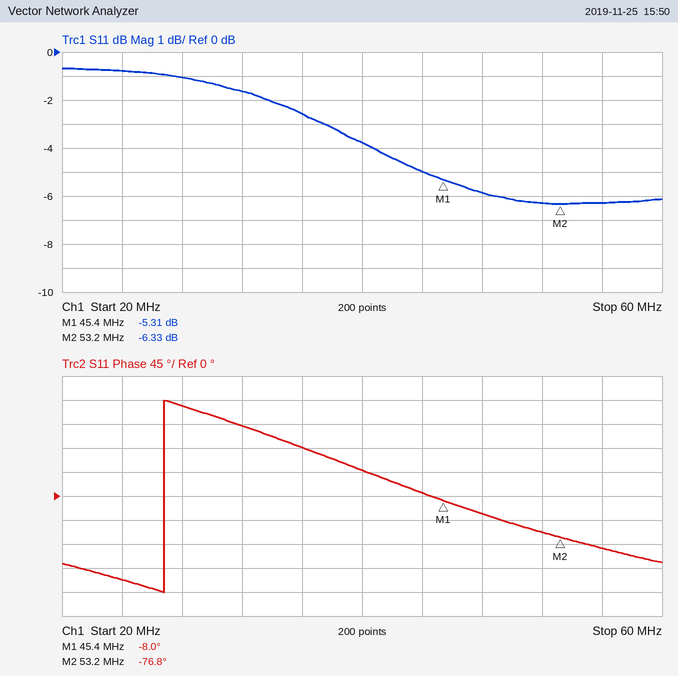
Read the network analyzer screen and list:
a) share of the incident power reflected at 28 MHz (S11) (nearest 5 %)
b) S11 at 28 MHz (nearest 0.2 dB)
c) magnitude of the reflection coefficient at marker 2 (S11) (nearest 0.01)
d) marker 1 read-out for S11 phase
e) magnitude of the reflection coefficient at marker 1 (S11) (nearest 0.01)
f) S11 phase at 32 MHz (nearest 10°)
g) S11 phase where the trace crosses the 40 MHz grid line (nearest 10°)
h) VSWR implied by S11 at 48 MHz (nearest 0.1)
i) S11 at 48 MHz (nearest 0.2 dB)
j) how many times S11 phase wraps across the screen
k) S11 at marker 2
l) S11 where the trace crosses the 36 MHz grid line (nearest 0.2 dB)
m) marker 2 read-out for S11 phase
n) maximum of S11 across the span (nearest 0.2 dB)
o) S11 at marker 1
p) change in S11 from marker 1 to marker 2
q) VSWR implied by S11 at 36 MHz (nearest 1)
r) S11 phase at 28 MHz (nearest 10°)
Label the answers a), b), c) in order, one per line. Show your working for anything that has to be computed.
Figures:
a) 10^(-1/10) ≈ 79.4 %, so 80 % to the nearest 5 %
b) -1.0 dB
c) 10^(-6.33/20) ≈ 0.48
d) -8.0°
e) 10^(-5.31/20) ≈ 0.54
f) 130°
g) 50°
h) |Γ| = 10^(-5.8/20) = 0.5129; VSWR = (1 + 0.5129)/(1 − 0.5129) ≈ 3.1
i) -5.8 dB
j) 1
k) -6.33 dB
l) -2.6 dB
m) -76.8°
n) -0.6 dB
o) -5.31 dB
p) -6.33 − (-5.31) = -1.02 dB
q) |Γ| = 10^(-2.6/20) = 0.7413; VSWR = (1 + 0.7413)/(1 − 0.7413) ≈ 7
r) 170°
